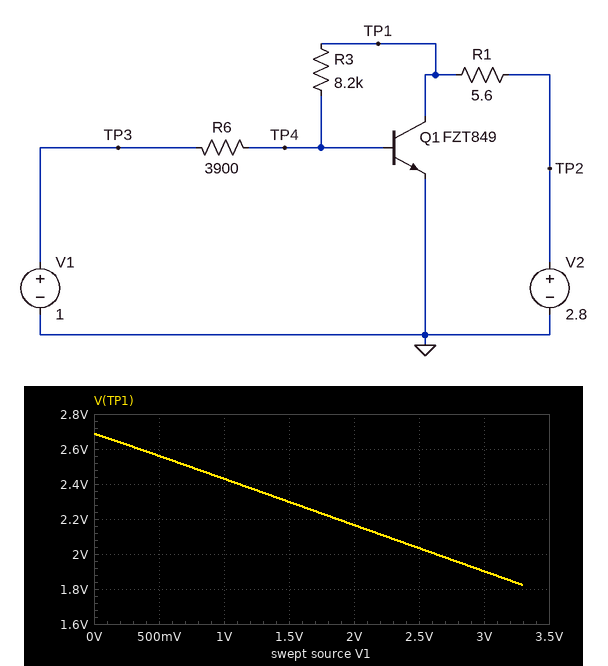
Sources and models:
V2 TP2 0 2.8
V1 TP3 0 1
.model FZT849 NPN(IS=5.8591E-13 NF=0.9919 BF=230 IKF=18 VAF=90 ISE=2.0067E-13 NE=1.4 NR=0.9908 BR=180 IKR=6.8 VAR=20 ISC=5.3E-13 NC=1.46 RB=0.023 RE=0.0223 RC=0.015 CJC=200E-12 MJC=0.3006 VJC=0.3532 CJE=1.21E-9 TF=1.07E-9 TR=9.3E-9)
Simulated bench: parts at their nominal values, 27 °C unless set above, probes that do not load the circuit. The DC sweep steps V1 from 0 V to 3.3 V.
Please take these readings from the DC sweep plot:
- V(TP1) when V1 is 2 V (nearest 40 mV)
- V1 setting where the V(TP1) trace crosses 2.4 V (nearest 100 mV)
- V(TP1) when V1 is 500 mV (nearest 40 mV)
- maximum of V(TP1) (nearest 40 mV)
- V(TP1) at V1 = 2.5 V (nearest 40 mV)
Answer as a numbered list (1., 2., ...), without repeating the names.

1. 2.16 V
2. 1.1 V
3. 2.56 V
4. 2.68 V
5. 2.04 V
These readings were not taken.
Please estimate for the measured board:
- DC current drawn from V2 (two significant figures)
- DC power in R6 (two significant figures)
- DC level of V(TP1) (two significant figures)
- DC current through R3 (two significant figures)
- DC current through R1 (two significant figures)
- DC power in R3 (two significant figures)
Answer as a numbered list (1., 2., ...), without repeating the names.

1. 66 mA
2. 31 µW
3. 2.4 V
4. 220 µA
5. 66 mA
6. 380 µW
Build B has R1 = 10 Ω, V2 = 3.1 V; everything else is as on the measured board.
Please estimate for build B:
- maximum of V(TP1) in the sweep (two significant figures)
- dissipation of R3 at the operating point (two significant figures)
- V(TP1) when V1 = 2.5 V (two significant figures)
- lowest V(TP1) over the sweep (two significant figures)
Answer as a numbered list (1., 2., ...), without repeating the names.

1. 2.9 V
2. 390 µW
3. 1.8 V
4. 1.5 V
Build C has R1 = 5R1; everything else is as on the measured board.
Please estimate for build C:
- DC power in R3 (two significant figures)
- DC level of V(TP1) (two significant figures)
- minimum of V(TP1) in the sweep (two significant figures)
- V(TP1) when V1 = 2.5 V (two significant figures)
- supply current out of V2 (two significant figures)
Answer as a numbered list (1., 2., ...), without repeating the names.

1. 400 µW
2. 2.5 V
3. 1.9 V
4. 2.1 V
5. 67 mA
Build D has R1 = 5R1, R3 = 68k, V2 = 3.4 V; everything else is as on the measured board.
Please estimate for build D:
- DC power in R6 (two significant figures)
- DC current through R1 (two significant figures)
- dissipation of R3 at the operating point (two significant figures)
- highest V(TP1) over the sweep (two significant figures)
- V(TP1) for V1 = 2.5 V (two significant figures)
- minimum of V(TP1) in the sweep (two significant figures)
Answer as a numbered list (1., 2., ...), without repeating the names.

1. 35 µW
2. 29 mA
3. 100 µW
4. 3.4 V
5. 2.8 V
6. 2.6 V
